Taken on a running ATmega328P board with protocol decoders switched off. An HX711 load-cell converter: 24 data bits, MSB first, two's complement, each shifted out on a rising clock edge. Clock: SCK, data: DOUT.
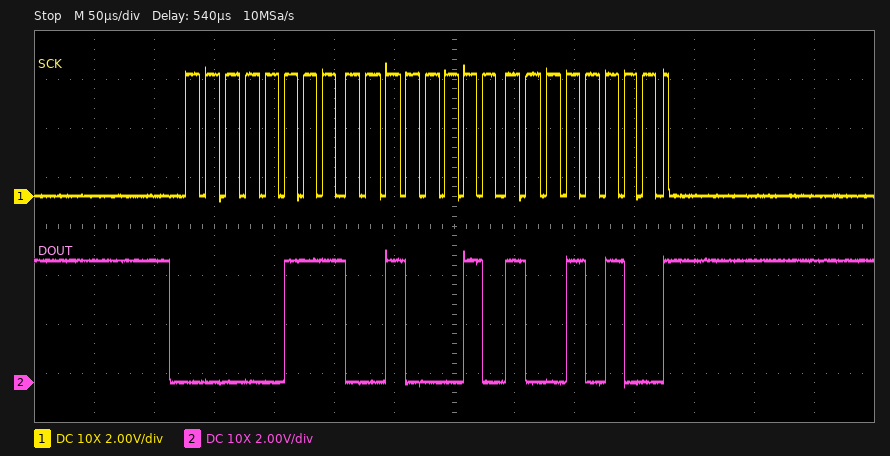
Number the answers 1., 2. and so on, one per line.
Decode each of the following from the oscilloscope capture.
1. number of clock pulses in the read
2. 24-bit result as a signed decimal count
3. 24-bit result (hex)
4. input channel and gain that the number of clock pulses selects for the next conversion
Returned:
1. 25
2. 467604
3. 0x072294
4. channel A, gain 128
